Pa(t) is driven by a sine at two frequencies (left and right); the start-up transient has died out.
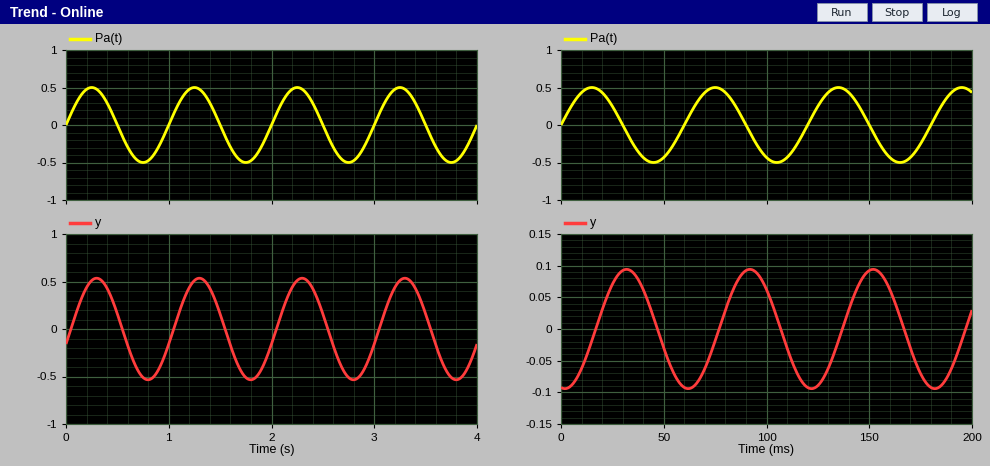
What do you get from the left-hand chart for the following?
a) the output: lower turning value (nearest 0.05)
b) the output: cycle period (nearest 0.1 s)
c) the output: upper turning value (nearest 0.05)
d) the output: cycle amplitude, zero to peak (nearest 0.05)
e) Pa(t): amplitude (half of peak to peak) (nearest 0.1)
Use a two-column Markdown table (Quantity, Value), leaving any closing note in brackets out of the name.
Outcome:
| Quantity | Value |
|---|---|
| the output: lower turning value | -0.55 |
| the output: cycle period | 1.0 s |
| the output: upper turning value | 0.55 |
| the output: cycle amplitude, zero to peak | 0.55 |
| Pa(t): amplitude (half of peak to peak) | 0.5 |
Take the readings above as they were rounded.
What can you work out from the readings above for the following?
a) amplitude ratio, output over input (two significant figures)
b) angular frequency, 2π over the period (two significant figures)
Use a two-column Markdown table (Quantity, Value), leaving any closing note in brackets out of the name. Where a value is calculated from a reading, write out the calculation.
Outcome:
| Quantity | Value |
|---|---|
| amplitude ratio, output over input | 0.55 / 0.5 = 1.1 |
| angular frequency, 2π over the period | 2π / 1 = 6.3 rad/s |
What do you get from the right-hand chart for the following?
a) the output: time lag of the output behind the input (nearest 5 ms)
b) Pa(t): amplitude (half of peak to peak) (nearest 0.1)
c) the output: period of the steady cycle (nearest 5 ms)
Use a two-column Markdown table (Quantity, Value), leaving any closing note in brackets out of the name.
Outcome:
| Quantity | Value |
|---|---|
| the output: time lag of the output behind the input | 15 ms |
| Pa(t): amplitude (half of peak to peak) | 0.5 |
| the output: period of the steady cycle | 60 ms |
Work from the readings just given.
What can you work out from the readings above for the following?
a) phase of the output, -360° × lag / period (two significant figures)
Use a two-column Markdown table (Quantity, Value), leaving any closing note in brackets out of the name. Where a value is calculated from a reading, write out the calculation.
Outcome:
| Quantity | Value |
|---|---|
| phase of the output, -360° × lag / period | -360 × 15 / 60 = -90° |
